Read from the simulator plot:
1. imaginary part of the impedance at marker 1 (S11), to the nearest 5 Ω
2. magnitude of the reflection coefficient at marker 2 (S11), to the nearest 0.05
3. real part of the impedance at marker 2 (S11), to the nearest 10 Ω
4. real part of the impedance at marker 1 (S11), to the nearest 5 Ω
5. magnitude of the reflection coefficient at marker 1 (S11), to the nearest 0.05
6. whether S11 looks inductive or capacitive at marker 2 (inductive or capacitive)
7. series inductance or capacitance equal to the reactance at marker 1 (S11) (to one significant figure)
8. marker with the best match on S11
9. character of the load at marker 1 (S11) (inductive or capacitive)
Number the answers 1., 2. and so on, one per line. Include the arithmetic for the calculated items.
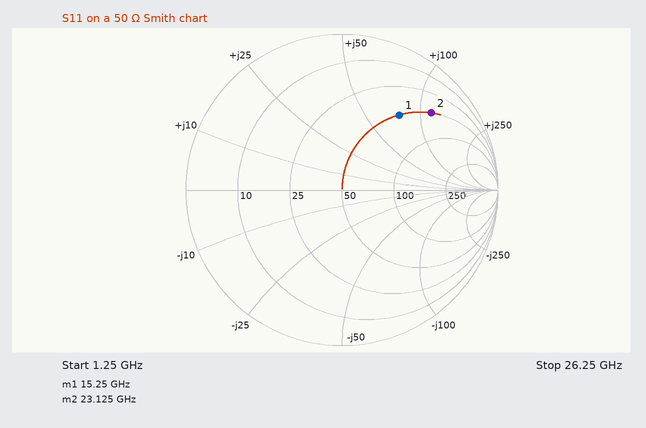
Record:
1. +75 Ω
2. 0.75
3. 50 Ω
4. 50 Ω
5. 0.60
6. inductive
7. L = 75 Ω/(2π × 15.25 GHz) ≈ 783 pH, so 800 pH to one significant figure
8. marker 1
9. inductive
